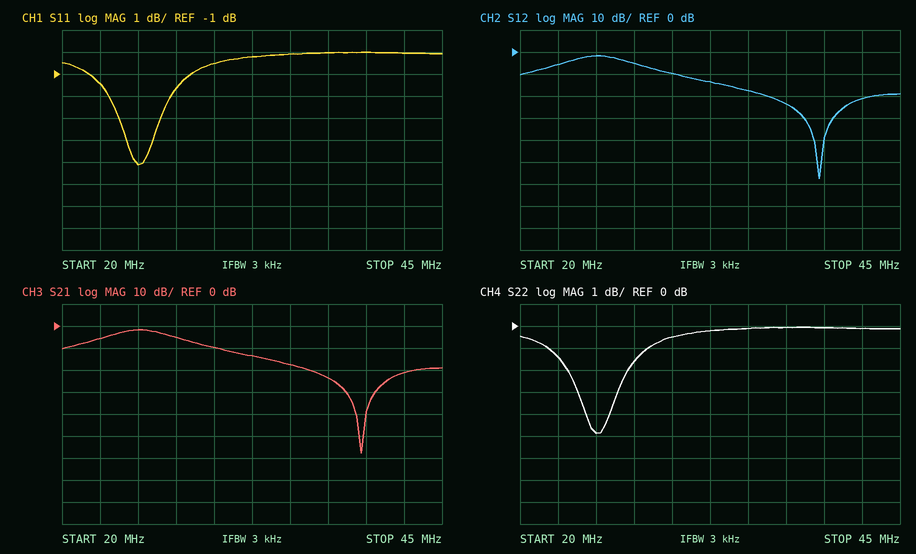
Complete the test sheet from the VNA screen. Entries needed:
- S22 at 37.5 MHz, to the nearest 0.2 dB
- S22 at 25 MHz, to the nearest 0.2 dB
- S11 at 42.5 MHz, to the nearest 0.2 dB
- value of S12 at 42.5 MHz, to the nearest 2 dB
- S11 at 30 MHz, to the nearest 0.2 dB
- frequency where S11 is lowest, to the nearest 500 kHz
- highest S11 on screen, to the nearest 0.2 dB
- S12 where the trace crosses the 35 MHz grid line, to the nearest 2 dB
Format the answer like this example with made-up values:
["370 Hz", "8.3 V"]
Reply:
["0.0 dB", "-4.8 dB", "0.0 dB", "-22 dB", "-0.6 dB", "25.0 MHz", "0.0 dB", "-18 dB"]
